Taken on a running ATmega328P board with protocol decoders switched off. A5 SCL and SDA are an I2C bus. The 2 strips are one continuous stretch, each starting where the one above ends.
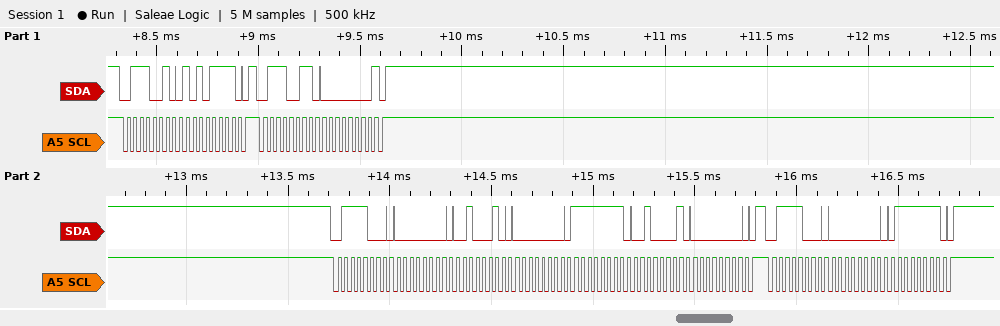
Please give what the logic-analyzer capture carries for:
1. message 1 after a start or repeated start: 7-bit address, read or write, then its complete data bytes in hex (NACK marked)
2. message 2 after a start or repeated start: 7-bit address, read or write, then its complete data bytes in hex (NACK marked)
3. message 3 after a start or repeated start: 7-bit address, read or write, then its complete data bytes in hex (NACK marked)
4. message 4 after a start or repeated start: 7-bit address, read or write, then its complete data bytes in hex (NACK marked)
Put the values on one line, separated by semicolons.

0x39 write: AF; 0x39 read: 00 NACK; 0x3C write: 00 22 00 FF 21 00; 0x3C write: 00 7F
